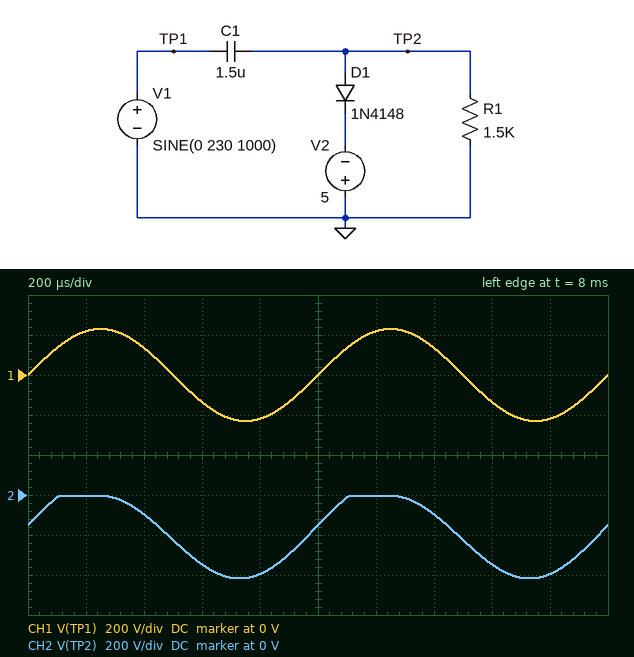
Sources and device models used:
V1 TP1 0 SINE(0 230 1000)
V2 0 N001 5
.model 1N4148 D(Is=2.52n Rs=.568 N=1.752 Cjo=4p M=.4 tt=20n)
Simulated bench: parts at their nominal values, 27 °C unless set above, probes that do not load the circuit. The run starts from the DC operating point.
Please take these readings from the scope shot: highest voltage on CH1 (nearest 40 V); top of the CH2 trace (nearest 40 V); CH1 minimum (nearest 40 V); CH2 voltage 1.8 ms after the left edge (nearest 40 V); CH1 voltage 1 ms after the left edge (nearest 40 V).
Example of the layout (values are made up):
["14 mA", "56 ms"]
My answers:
["240 V", "0 V", "-240 V", "-400 V", "0 V"]
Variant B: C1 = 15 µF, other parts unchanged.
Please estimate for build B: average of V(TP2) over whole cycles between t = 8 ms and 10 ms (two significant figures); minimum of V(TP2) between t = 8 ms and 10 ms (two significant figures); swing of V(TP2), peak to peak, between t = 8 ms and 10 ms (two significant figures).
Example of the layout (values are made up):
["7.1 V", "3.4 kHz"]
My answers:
["-230 V", "-460 V", "460 V"]
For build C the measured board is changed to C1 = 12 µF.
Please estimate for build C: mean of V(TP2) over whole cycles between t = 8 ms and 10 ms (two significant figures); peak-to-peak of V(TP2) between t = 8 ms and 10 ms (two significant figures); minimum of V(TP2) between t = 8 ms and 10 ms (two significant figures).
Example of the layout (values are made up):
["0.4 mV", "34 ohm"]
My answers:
["-230 V", "460 V", "-460 V"]
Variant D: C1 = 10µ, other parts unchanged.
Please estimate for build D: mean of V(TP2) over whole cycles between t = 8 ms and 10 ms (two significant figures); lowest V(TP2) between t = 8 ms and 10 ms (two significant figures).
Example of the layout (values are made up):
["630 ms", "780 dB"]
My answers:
["-230 V", "-460 V"]
